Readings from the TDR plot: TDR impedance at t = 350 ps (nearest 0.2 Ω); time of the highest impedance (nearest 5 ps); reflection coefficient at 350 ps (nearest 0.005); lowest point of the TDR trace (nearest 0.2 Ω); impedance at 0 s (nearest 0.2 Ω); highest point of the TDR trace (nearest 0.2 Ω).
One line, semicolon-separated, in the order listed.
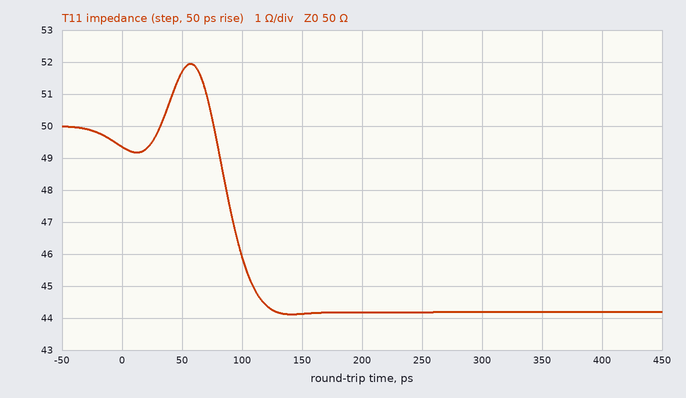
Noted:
44.2 Ω; 55 ps; -0.060; 44.2 Ω; 49.4 Ω; 52.0 Ω
